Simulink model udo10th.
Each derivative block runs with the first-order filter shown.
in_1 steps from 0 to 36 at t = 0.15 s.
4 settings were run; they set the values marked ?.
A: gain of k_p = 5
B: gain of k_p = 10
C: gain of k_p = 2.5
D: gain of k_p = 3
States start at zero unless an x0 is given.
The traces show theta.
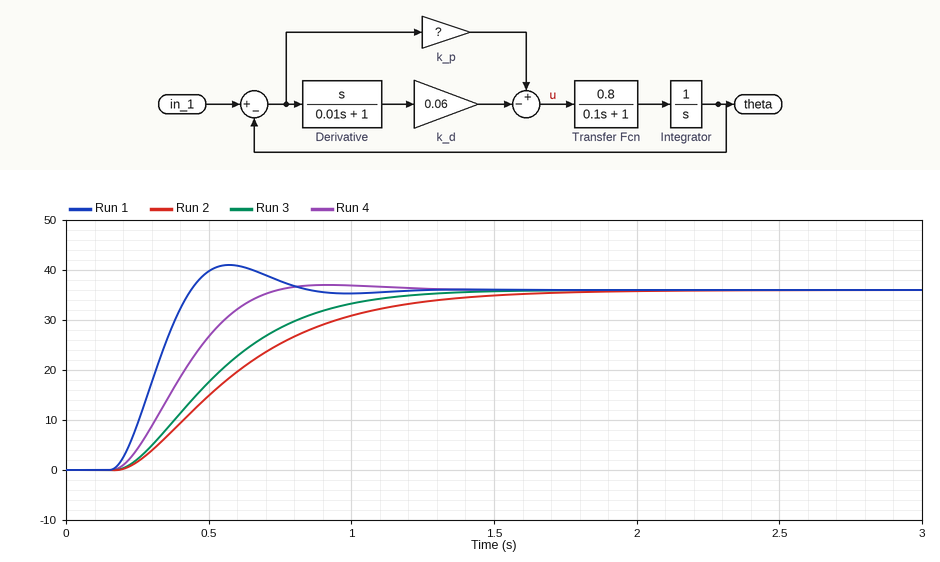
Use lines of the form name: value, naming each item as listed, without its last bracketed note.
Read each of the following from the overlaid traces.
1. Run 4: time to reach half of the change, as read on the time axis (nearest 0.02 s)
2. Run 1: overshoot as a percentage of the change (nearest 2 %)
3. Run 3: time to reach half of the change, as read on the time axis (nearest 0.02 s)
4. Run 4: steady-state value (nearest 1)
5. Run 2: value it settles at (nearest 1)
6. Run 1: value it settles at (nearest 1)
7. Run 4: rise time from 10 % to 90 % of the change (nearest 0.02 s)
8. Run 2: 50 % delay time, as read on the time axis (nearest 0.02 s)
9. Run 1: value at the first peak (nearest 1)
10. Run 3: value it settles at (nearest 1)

Run 4: time to reach half of the change, as read on the time axis: 0.40 s
Run 1: overshoot as a percentage of the change: 14 %
Run 3: time to reach half of the change, as read on the time axis: 0.50 s
Run 4: steady-state value: 36
Run 2: value it settles at: 36
Run 1: value it settles at: 36
Run 4: rise time from 10 % to 90 % of the change: 0.36 s
Run 2: 50 % delay time, as read on the time axis: 0.56 s
Run 1: value at the first peak: 41
Run 3: value it settles at: 36
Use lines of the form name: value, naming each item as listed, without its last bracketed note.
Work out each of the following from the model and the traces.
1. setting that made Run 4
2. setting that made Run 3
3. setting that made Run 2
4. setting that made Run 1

setting that made Run 4: A
setting that made Run 3: D
setting that made Run 2: C
setting that made Run 1: B
